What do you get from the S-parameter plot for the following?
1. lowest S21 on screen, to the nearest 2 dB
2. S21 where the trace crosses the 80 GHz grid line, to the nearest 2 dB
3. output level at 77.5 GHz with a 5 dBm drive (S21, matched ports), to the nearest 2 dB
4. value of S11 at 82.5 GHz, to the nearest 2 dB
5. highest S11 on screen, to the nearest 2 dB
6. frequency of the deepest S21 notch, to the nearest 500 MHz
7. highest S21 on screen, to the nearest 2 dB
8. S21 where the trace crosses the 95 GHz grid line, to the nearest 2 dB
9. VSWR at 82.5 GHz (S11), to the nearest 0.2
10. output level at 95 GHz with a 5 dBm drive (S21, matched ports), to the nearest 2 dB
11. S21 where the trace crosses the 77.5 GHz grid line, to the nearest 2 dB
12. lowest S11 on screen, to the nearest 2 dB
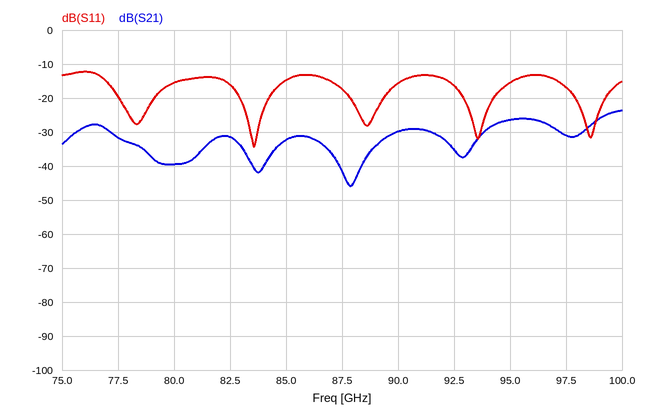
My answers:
-46 dB
-40 dB
-26 dBm
-16 dB
-12 dB
88.0 GHz
-24 dB
-26 dB
1.4
-22 dBm
-32 dB
-34 dB
